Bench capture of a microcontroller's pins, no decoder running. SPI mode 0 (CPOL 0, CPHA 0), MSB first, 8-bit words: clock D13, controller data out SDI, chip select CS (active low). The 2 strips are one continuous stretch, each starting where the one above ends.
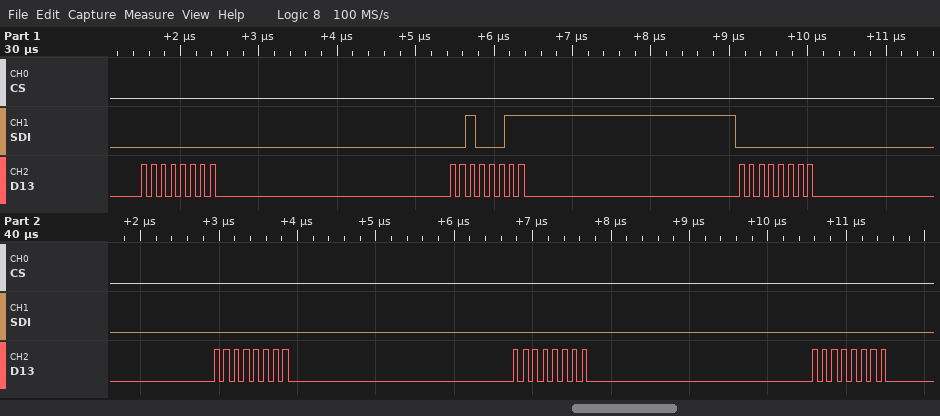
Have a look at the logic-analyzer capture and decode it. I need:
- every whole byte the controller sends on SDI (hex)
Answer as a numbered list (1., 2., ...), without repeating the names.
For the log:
1. 0x00 0x23 0x00 0x00 0x00 0x00
